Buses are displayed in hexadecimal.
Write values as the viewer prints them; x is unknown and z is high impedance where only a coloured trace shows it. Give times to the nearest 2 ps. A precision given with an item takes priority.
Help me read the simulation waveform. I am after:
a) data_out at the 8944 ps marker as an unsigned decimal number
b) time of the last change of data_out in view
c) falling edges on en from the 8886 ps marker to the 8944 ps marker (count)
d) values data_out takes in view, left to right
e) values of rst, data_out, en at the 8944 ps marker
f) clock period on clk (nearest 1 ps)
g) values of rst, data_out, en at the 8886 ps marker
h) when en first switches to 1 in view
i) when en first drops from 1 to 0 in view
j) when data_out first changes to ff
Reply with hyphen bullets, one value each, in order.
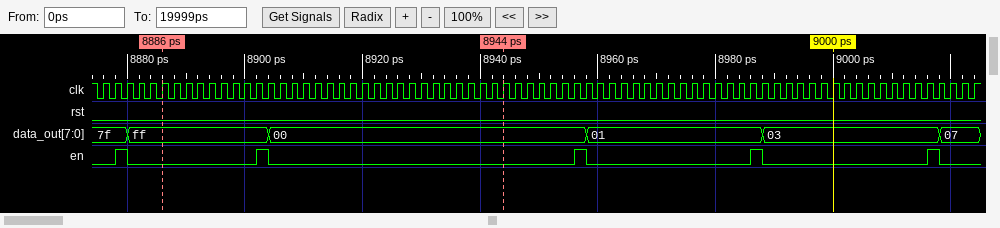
- 0
- 9018 ps
- 1
- 7f, ff, 00, 01, 03, 07
- rst=0, data_out=00, en=0
- 2 ps
- rst=0, data_out=ff, en=0
- 8878 ps
- 8880 ps
- 8880 ps
